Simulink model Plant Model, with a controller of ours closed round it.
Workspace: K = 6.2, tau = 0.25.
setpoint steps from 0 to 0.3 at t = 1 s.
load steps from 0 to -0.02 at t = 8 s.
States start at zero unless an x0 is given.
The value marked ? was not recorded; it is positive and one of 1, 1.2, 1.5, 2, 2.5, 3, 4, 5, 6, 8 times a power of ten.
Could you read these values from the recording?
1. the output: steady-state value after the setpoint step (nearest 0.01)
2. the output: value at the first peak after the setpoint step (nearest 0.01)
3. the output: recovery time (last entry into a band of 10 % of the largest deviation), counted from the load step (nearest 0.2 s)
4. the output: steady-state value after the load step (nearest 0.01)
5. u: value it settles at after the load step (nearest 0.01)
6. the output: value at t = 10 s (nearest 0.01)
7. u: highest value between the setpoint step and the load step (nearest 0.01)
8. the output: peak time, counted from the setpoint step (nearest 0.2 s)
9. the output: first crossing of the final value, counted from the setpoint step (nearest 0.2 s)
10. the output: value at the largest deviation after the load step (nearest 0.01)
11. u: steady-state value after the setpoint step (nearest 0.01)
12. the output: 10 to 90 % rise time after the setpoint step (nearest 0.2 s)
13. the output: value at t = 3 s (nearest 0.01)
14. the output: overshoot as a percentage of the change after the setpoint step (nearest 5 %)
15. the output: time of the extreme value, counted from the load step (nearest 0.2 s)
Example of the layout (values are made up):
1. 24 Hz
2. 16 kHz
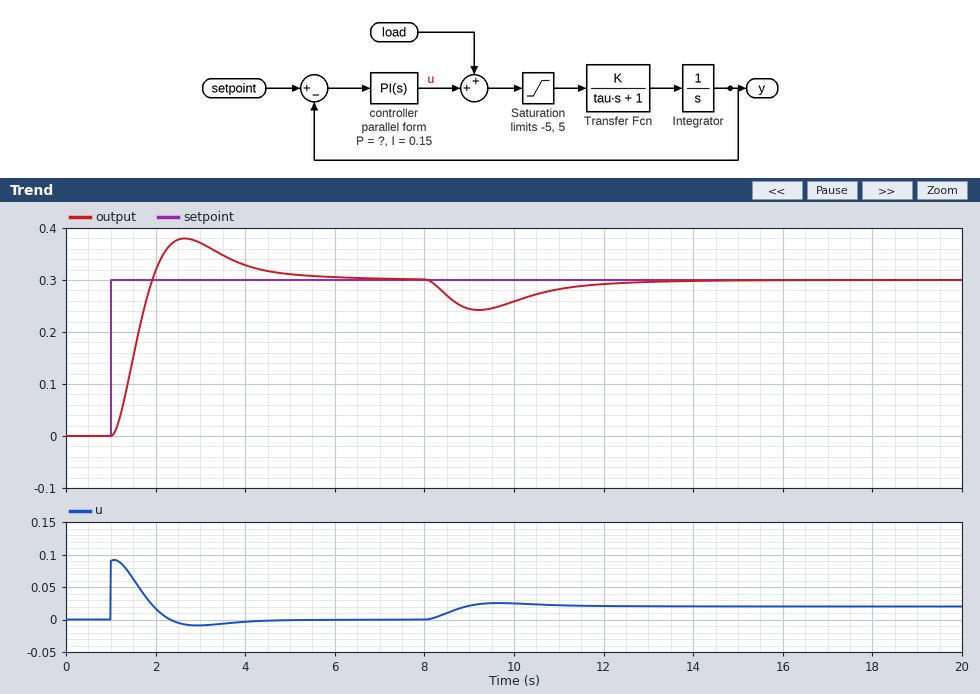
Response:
1. 0.30
2. 0.38
3. 4.4 s
4. 0.30
5. 0.02
6. 0.26
7. 0.09
8. 1.6 s
9. 1.0 s
10. 0.24
11. 0.00
12. 0.6 s
13. 0.37
14. 25 %
15. 1.2 s
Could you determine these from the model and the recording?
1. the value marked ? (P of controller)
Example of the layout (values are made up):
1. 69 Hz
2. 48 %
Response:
1. 0.3
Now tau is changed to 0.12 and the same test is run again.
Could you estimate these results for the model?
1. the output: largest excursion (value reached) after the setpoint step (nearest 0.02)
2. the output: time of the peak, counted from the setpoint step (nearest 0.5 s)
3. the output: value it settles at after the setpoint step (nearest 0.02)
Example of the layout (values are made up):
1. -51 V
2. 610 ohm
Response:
1. 0.36
2. 2.0 s
3. 0.30
